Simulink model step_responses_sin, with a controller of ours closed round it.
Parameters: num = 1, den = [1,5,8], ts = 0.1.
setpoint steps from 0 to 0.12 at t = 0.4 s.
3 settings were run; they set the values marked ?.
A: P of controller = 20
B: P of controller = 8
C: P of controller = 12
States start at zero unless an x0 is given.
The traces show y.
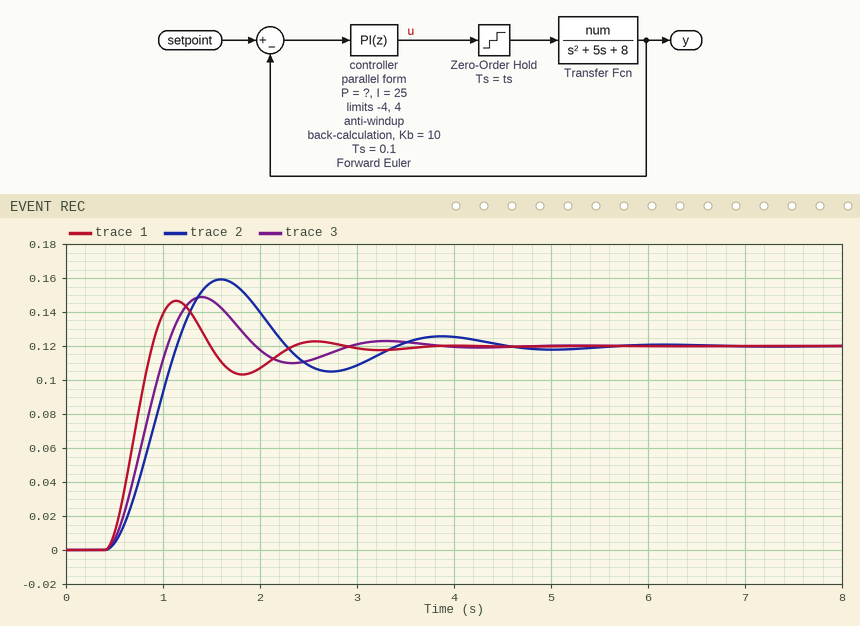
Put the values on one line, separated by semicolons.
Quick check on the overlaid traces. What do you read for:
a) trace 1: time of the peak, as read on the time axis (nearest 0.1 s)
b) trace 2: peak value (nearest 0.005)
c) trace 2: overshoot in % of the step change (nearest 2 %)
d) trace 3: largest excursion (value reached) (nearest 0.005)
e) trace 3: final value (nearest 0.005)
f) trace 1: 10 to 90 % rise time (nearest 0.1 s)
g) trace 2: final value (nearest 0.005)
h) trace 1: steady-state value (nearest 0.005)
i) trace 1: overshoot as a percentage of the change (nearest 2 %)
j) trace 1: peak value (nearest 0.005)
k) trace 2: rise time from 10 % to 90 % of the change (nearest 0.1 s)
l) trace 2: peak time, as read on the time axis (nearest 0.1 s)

1.1 s; 0.160; 32 %; 0.150; 0.120; 0.3 s; 0.120; 0.120; 22 %; 0.145; 0.5 s; 1.6 s
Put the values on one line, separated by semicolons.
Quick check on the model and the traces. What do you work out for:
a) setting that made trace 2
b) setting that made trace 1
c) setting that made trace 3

B; A; C
